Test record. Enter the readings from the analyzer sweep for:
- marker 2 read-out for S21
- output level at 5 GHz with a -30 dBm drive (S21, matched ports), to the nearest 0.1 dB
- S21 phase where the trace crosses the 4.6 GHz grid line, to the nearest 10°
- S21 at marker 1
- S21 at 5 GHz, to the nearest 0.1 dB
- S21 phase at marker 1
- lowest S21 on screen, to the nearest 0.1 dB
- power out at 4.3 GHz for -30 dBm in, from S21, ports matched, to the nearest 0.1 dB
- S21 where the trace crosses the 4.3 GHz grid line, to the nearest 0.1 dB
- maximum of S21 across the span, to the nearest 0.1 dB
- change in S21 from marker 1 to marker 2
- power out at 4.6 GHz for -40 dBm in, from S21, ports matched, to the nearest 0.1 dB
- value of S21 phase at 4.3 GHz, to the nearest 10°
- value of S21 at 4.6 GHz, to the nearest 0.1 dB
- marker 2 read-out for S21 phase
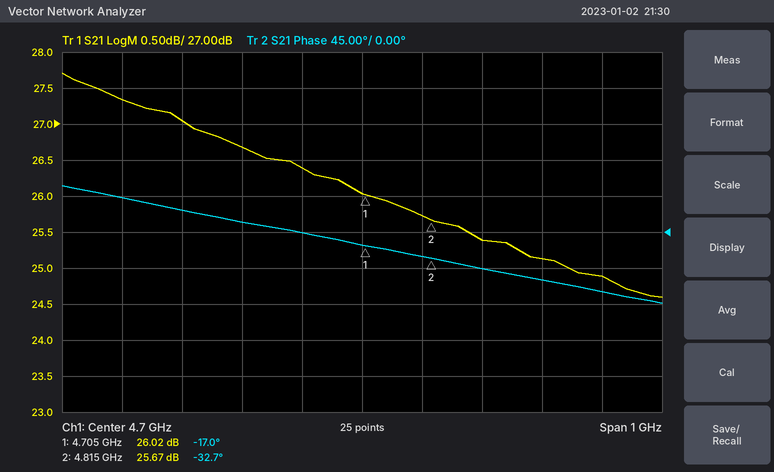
25.67 dB
-4.9 dBm
0°
26.02 dB
25.1 dB
-17.0°
24.6 dB
-2.7 dBm
27.3 dB
27.7 dB
-0.35 dB
-13.6 dBm
40°
26.4 dB
-32.7°
